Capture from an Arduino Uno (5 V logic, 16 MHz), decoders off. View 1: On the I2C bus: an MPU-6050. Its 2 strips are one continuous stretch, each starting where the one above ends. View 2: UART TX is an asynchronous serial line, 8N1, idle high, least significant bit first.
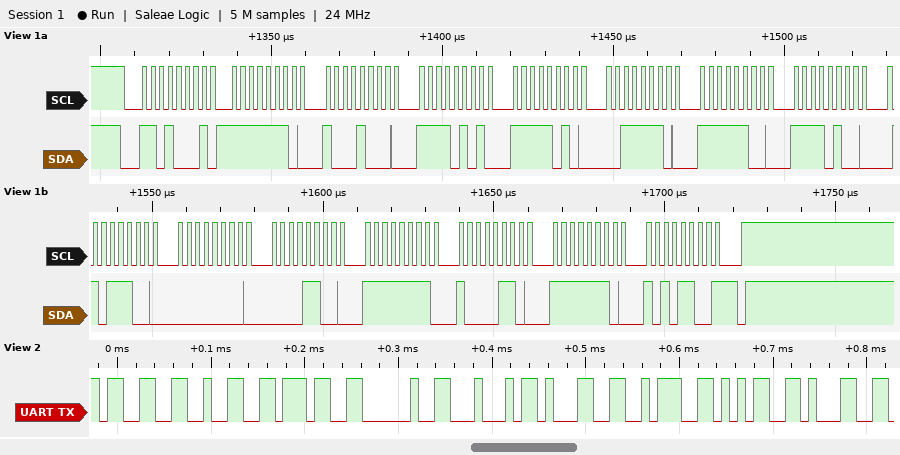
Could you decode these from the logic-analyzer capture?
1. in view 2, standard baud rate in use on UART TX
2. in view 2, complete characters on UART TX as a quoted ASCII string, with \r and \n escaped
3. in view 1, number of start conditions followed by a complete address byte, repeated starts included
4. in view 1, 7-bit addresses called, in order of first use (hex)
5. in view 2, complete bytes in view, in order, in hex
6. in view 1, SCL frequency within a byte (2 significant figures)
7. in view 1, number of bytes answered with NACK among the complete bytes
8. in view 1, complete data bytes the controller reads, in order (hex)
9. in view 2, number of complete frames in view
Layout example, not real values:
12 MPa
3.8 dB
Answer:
115200 baud
"327 D1:51"
1
0x68
33 32 37 20 44 31 3A 35 31
400 kHz
1
FE 88 F5 FA 3E FC F4 5C 00 0C FF 86 FE AC
9
